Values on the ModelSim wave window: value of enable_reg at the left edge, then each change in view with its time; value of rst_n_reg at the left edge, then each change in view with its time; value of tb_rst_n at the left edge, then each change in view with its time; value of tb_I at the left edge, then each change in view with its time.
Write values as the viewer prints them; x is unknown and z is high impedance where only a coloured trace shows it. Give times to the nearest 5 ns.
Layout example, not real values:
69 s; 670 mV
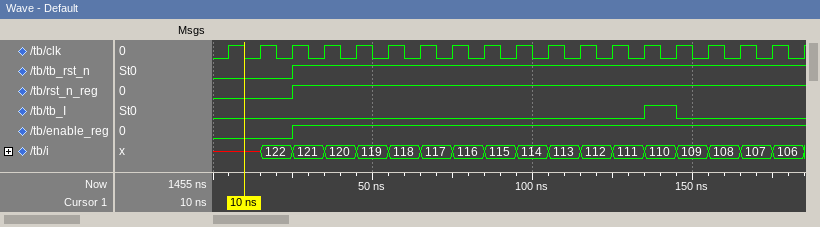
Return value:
0, 1 at 25 ns; 0, 1 at 25 ns; 0, 1 at 25 ns; 0, 1 at 135 ns, 0 at 145 ns
